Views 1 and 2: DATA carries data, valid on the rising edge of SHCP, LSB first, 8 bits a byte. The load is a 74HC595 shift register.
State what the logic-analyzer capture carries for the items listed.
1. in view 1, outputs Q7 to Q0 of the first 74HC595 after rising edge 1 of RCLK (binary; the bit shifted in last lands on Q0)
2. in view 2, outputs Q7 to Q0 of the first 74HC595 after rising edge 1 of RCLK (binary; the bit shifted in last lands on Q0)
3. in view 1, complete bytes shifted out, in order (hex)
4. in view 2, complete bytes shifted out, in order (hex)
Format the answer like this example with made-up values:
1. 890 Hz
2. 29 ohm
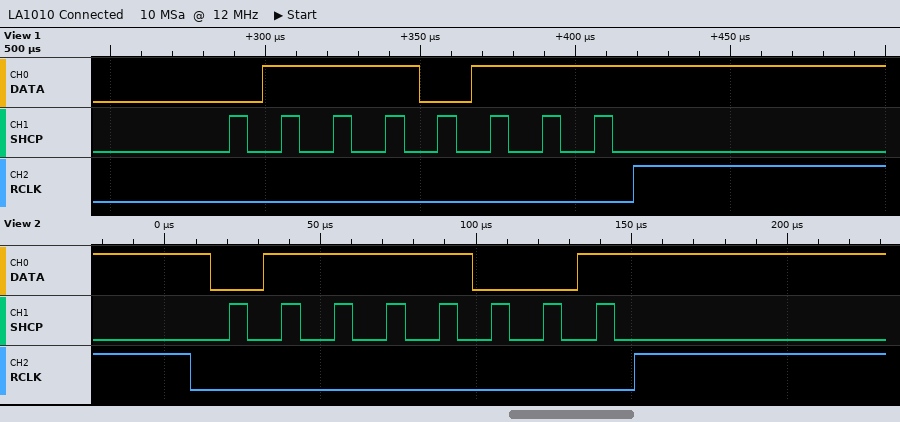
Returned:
1. 01110111
2. 01111001
3. EE
4. 9E
